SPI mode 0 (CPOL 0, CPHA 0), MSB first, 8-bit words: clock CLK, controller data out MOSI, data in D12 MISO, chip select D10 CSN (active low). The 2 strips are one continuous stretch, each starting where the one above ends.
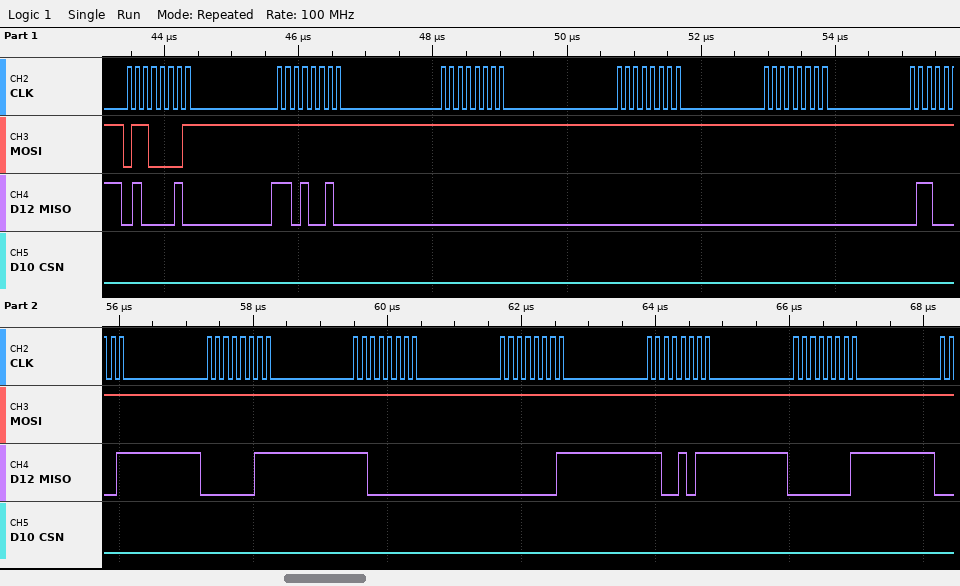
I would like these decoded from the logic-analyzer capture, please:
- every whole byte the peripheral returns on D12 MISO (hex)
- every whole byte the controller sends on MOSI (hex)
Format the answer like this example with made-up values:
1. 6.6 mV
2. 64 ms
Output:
1. 0x42 0xD2 0x00 0x00 0x00 0x61 0x03 0xC0 0x01 0xCB 0x01
2. 0x61 0xFF 0xFF 0xFF 0xFF 0xFF 0xFF 0xFF 0xFF 0xFF 0xFF
